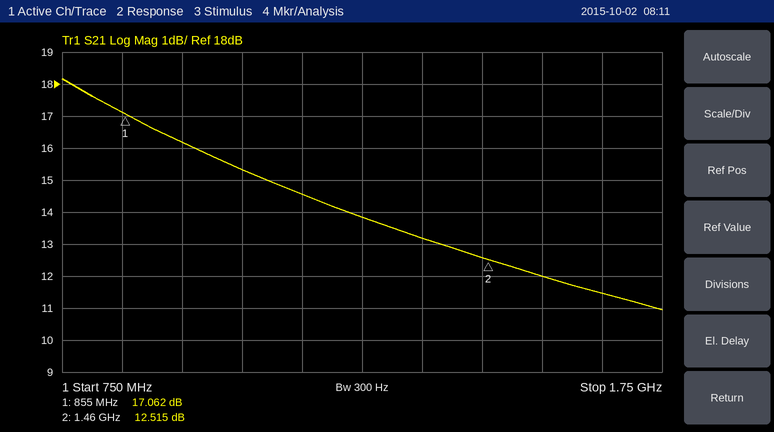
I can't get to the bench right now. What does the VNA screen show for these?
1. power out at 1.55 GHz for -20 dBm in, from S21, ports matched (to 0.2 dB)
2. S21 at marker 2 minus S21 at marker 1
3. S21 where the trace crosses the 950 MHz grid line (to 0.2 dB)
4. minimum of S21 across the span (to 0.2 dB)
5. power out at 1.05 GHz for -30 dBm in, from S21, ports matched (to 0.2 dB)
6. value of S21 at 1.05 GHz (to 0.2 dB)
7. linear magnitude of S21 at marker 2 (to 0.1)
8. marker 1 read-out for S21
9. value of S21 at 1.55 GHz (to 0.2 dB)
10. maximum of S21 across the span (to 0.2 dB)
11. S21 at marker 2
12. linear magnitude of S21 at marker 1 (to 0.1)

-8.0 dBm
-4.547 dB
16.2 dB
11.0 dB
-14.6 dBm
15.4 dB
4.2
17.062 dB
12.0 dB
18.2 dB
12.515 dB
7.1
